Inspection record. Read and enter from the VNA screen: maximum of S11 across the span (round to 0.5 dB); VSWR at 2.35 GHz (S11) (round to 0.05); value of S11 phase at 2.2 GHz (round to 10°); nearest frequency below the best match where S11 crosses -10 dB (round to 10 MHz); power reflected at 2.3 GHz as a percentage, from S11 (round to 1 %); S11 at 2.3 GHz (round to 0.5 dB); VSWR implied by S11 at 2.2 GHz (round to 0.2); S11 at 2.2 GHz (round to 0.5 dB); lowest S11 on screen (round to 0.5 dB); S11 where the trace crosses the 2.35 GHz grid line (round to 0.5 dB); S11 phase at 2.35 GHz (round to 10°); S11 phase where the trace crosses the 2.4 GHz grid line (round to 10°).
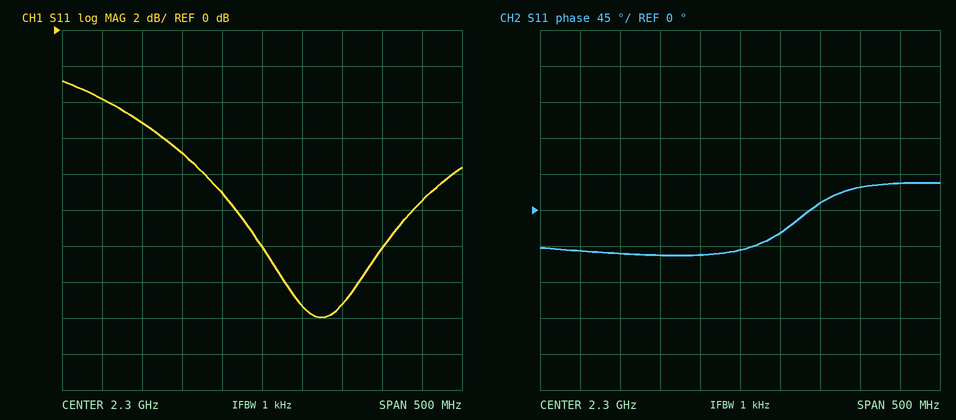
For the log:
-3.0 dB
1.40
-60°
2.27 GHz
6 %
-12.0 dB
2.6
-7.0 dB
-16.0 dB
-15.5 dB
-30°
10°
